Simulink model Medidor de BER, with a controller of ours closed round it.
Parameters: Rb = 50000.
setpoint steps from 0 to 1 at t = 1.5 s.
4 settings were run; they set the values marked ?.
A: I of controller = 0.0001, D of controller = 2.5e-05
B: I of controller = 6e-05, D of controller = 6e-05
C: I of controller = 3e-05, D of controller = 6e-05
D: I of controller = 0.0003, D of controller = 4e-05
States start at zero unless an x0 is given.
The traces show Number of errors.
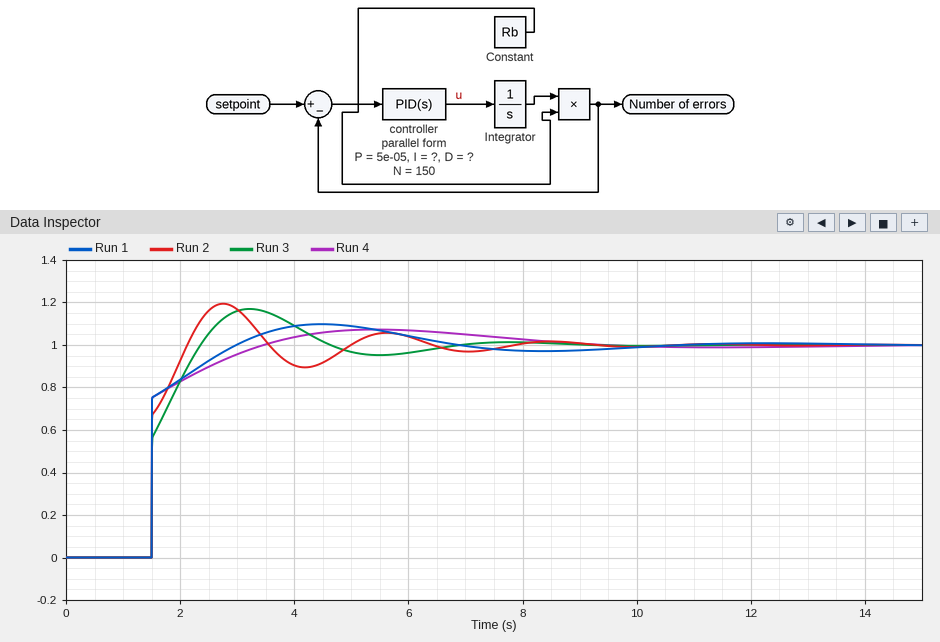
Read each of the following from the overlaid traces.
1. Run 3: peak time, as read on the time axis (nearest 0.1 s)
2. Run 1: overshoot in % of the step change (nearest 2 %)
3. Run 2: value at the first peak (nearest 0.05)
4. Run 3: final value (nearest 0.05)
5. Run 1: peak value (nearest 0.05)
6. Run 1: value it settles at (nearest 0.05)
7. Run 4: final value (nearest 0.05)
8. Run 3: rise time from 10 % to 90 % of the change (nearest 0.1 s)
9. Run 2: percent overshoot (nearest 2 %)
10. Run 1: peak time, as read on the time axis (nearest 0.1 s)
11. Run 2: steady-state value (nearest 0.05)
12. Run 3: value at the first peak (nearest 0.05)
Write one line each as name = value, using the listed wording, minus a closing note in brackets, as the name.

Run 3: peak time, as read on the time axis = 3.2 s
Run 1: overshoot in % of the step change = 10 %
Run 2: value at the first peak = 1.20
Run 3: final value = 1.00
Run 1: peak value = 1.10
Run 1: value it settles at = 1.00
Run 4: final value = 1.00
Run 3: rise time from 10 % to 90 % of the change = 0.6 s
Run 2: percent overshoot = 20 %
Run 1: peak time, as read on the time axis = 4.5 s
Run 2: steady-state value = 1.00
Run 3: value at the first peak = 1.15
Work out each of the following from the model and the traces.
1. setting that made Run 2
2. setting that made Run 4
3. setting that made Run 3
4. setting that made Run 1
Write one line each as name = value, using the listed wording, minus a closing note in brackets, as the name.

setting that made Run 2 = D
setting that made Run 4 = C
setting that made Run 3 = A
setting that made Run 1 = B
